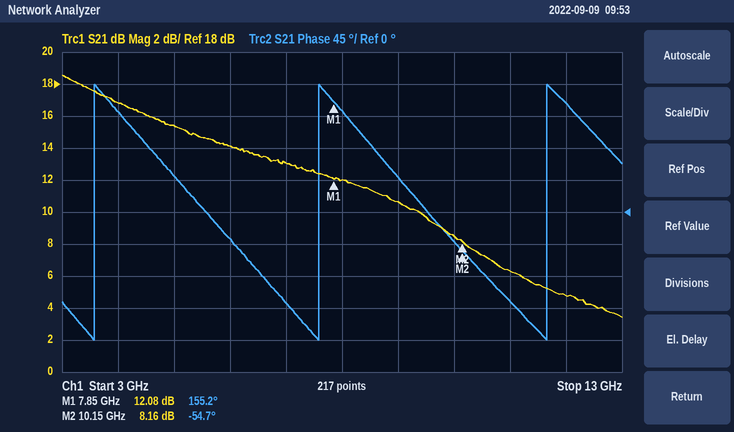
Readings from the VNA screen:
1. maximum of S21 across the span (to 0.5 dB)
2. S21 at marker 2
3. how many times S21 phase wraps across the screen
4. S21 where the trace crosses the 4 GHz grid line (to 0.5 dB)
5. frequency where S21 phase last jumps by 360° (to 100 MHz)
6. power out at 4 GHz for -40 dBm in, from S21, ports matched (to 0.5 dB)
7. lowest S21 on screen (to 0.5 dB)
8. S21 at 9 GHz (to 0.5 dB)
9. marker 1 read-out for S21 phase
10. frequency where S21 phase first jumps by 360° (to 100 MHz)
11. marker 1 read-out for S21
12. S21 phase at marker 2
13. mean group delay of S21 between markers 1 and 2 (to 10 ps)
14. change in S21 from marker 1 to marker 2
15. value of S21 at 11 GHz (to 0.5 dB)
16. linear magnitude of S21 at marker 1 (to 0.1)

18.5 dB
8.16 dB
3
17.0 dB
11.7 GHz
-23.0 dBm
3.5 dB
10.5 dB
155.2°
3.6 GHz
12.08 dB
-54.7°
250 ps
-3.92 dB
6.5 dB
4.0
